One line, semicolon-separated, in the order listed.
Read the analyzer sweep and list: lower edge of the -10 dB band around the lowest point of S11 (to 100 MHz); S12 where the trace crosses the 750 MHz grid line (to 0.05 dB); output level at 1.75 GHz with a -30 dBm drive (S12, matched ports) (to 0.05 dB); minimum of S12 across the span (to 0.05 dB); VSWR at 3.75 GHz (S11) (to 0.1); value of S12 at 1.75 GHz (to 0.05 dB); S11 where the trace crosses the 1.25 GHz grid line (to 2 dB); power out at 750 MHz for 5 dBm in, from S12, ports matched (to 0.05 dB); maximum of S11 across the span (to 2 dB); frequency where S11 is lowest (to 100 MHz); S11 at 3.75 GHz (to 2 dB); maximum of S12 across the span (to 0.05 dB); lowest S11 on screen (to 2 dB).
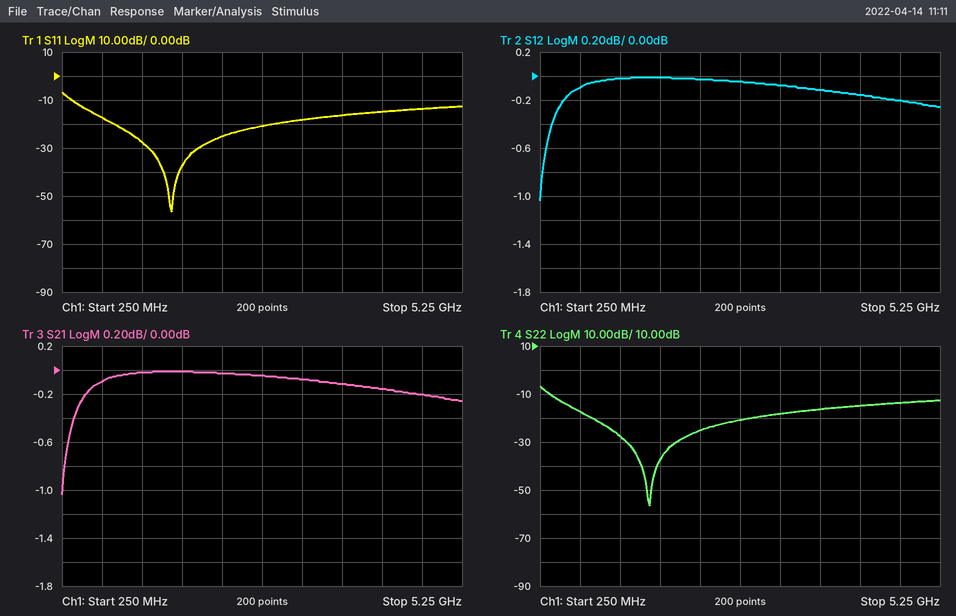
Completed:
400 MHz; -0.10 dB; -30.00 dBm; -1.05 dB; 1.4; 0.00 dB; -28 dB; 4.90 dBm; -6 dB; 1.6 GHz; -16 dB; 0.00 dB; -56 dB
